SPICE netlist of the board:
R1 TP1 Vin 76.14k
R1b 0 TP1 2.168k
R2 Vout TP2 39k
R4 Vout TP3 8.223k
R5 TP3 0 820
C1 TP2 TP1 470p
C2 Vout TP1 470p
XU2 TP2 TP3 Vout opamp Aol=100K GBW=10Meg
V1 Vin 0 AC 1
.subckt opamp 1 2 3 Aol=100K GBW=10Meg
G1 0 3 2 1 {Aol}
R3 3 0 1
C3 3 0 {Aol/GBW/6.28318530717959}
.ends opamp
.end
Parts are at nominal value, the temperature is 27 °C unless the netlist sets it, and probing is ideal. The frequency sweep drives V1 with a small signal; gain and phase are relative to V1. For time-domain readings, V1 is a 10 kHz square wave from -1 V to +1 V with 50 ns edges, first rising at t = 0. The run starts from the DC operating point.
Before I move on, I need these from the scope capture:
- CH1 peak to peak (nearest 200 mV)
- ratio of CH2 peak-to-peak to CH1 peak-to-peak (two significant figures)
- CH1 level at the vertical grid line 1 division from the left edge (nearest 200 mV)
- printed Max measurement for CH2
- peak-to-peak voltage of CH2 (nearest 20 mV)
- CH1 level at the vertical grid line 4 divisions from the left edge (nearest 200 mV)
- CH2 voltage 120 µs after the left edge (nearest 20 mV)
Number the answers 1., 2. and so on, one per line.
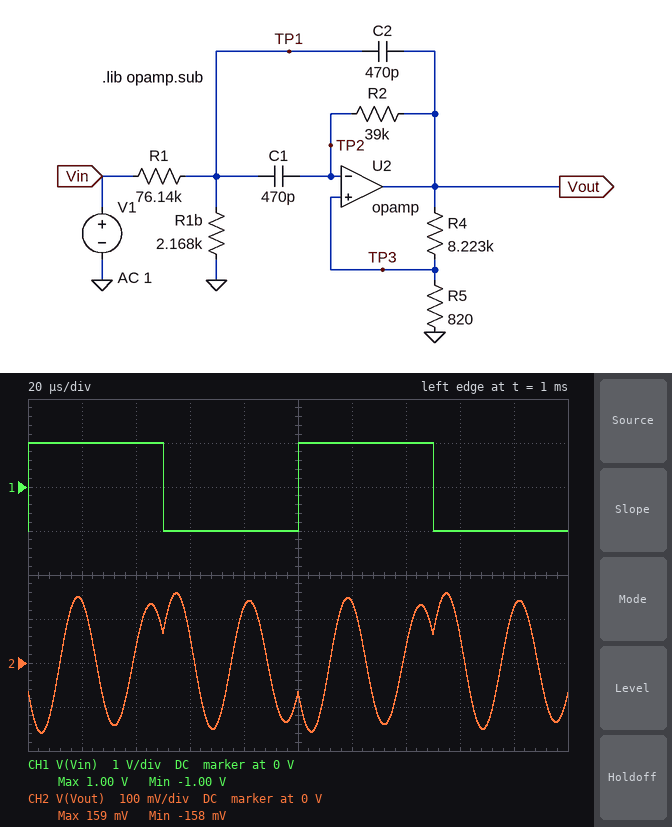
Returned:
1. 2.0 V
2. 0.16
3. 1.0 V
4. 159 mV
5. 320 mV
6. -1.0 V
7. 140 mV
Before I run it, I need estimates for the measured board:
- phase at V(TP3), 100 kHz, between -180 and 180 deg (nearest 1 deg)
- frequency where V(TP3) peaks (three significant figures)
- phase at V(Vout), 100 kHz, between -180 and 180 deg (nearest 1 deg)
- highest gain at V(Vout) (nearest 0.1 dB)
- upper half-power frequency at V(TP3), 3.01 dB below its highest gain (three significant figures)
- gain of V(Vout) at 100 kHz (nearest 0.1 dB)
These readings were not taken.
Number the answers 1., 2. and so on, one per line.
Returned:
1. 90 deg
2. 37.0 kHz
3. 90 deg
4. 11.2 dB
5. 37.7 kHz
6. -25.1 dB
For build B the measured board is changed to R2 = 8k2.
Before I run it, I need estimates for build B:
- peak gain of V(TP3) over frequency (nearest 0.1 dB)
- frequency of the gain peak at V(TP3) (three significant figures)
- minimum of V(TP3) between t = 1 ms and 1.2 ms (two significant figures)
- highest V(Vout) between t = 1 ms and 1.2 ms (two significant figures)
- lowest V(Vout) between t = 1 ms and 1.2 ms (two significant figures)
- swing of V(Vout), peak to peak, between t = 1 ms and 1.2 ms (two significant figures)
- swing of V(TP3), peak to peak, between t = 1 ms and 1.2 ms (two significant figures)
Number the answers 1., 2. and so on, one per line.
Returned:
1. -43.5 dB
2. 80.7 kHz
3. -6.5 mV
4. 71 mV
5. -71 mV
6. 140 mV
7. 13 mV
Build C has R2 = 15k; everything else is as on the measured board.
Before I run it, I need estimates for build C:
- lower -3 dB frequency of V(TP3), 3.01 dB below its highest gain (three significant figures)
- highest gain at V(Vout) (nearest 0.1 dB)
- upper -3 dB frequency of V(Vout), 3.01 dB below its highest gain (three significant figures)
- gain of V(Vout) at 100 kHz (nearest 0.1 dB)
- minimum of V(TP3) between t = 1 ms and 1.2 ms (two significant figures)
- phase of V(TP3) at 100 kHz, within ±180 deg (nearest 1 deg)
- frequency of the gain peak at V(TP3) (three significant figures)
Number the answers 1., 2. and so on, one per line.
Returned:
1. 47.0 kHz
2. -15.5 dB
3. 75.6 kHz
4. -23.3 dB
5. -10 mV
6. 113 deg
7. 59.6 kHz
